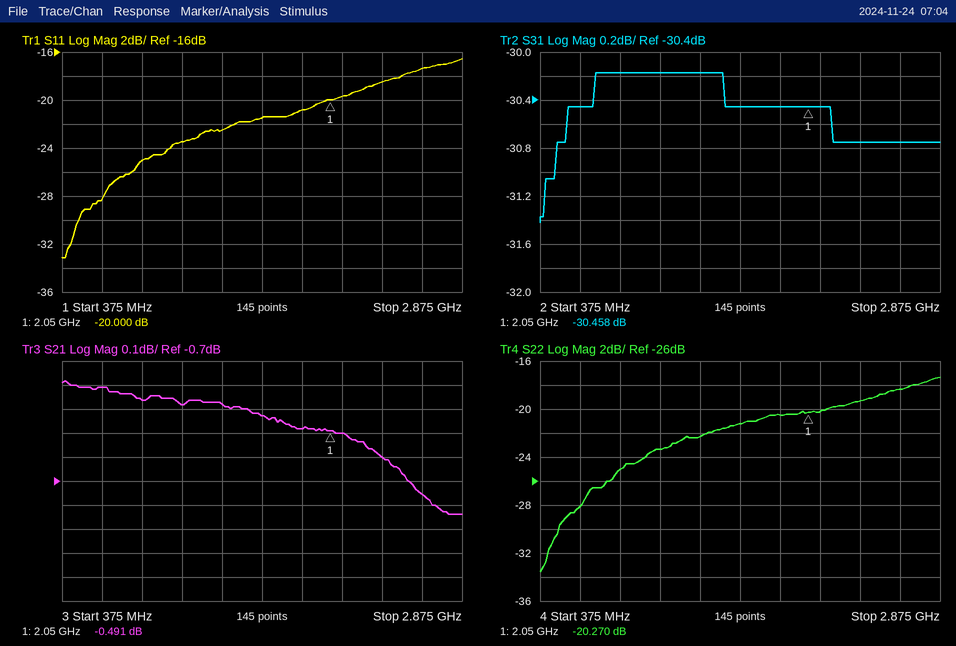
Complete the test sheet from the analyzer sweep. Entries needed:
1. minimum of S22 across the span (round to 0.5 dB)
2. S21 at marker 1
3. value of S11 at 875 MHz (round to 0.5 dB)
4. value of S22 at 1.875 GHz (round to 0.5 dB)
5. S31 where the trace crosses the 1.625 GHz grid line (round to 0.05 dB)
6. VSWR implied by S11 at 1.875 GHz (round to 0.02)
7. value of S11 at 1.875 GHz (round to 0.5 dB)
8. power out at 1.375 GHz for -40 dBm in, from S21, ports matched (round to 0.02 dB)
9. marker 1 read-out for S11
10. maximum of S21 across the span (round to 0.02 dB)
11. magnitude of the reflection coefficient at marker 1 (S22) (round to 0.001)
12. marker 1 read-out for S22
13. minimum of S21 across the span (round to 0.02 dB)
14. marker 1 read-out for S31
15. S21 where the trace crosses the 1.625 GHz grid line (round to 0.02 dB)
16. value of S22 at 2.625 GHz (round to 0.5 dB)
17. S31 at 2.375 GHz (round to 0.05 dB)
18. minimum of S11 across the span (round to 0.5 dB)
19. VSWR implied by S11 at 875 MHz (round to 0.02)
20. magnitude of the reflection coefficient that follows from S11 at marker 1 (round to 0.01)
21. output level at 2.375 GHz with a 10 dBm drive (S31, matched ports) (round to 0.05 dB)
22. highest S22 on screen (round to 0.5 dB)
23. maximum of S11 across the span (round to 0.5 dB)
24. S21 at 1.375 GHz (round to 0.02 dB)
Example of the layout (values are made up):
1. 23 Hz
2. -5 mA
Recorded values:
1. -33.5 dB
2. -0.491 dB
3. -25.0 dB
4. -20.5 dB
5. -30.45 dB
6. 1.20
7. -21.0 dB
8. -40.38 dBm
9. -20.000 dB
10. -0.28 dB
11. 0.097
12. -20.270 dB
13. -0.84 dB
14. -30.458 dB
15. -0.42 dB
16. -18.5 dB
17. -30.75 dB
18. -33.0 dB
19. 1.12
20. 0.10
21. -20.75 dBm
22. -17.5 dB
23. -16.5 dB
24. -0.38 dB
